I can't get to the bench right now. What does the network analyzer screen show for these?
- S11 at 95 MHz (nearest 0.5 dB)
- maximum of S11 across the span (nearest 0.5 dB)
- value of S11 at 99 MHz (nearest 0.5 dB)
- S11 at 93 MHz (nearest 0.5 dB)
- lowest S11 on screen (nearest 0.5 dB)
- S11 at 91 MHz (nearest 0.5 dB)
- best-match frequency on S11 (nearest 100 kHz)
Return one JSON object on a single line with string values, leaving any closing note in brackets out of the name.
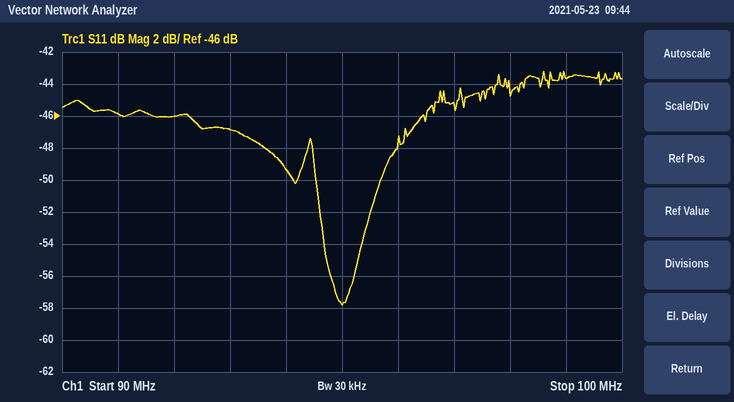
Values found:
{"S11 at 95 MHz": "-58.0 dB", "maximum of S11 across the span": "-43.0 dB", "value of S11 at 99 MHz": "-43.5 dB", "S11 at 93 MHz": "-47.0 dB", "lowest S11 on screen": "-58.0 dB", "S11 at 91 MHz": "-46.0 dB", "best-match frequency on S11": "95.0 MHz"}
